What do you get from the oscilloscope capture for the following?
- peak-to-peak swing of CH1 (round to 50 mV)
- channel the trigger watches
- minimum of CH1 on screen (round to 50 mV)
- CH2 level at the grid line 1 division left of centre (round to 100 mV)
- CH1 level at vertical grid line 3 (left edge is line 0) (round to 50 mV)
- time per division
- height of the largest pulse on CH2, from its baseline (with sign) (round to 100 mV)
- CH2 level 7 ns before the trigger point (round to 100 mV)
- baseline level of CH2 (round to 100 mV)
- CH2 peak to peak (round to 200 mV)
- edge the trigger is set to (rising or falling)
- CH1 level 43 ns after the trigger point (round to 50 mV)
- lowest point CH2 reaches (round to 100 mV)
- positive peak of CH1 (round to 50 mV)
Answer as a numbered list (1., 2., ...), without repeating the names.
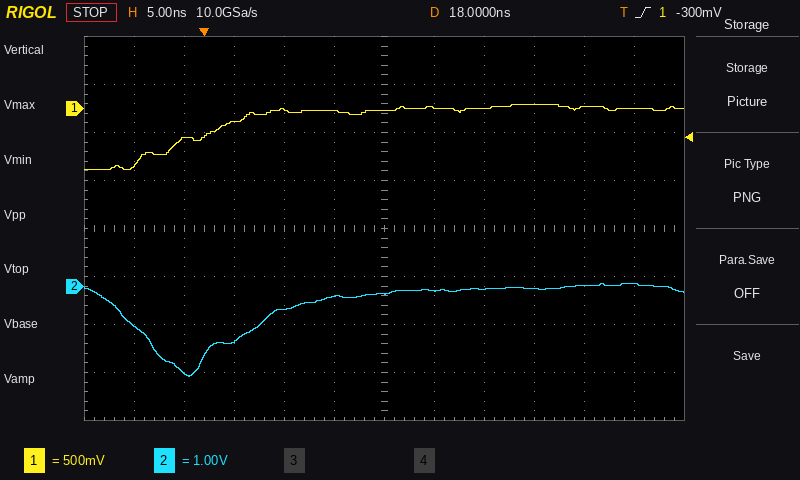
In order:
1. 700 mV
2. CH1
3. -650 mV
4. -200 mV
5. -150 mV
6. 5 ns
7. -1.8 V
8. -800 mV
9. -100 mV
10. 2.0 V
11. rising
12. 0 mV
13. -1.9 V
14. 50 mV
